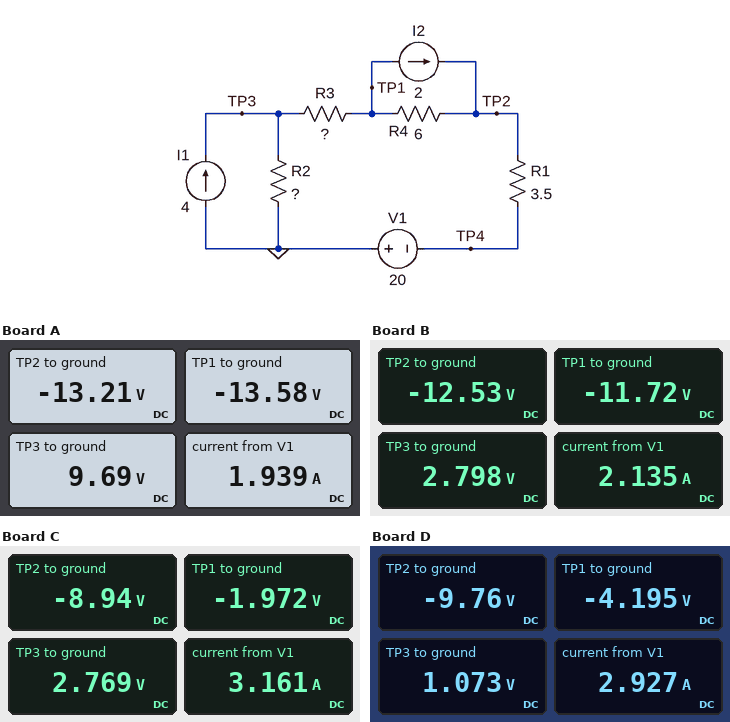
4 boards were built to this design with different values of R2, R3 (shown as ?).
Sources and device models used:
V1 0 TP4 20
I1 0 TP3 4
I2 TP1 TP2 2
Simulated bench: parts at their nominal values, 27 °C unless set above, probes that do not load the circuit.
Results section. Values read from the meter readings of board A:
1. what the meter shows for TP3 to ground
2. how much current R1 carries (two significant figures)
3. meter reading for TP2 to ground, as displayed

9.69 V
1.9 A
-13.21 V
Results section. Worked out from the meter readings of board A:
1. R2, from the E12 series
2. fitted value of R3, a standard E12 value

4.7 Ω
12 Ω
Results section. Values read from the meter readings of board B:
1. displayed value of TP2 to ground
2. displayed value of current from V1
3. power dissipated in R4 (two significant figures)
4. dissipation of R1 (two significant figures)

-12.53 V
2.135 A
110 mW
16 W
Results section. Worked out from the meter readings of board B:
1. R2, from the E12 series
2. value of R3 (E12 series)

1.5 Ω
6.8 Ω
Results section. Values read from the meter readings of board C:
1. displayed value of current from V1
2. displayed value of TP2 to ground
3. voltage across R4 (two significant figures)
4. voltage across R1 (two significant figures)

3.161 A
-8.94 V
7.0 V
11 V
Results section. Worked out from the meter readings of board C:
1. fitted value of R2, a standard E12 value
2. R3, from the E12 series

3.3 Ω
1.5 Ω
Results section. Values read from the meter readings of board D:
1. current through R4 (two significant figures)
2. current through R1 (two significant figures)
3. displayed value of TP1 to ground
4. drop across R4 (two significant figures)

930 mA
2.9 A
-4.195 V
5.6 V
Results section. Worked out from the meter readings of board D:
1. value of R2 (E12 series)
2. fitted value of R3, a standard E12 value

1 Ω
1.8 Ω
